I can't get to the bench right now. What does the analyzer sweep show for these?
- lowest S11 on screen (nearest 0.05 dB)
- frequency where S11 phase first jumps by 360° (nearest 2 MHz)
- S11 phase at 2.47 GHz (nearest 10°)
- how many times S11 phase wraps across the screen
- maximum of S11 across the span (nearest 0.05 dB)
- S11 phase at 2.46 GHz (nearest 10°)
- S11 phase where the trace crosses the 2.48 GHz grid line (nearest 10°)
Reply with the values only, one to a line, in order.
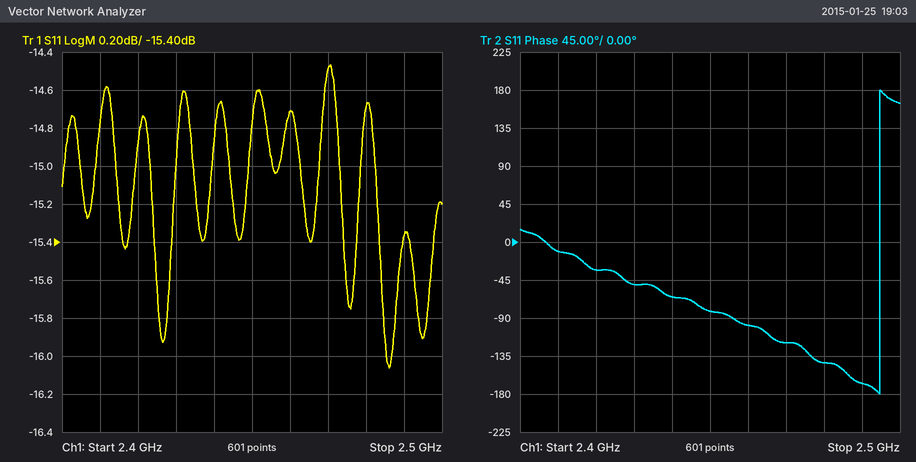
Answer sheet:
-16.05 dB
2.494 GHz
-120°
1
-14.45 dB
-100°
-140°
